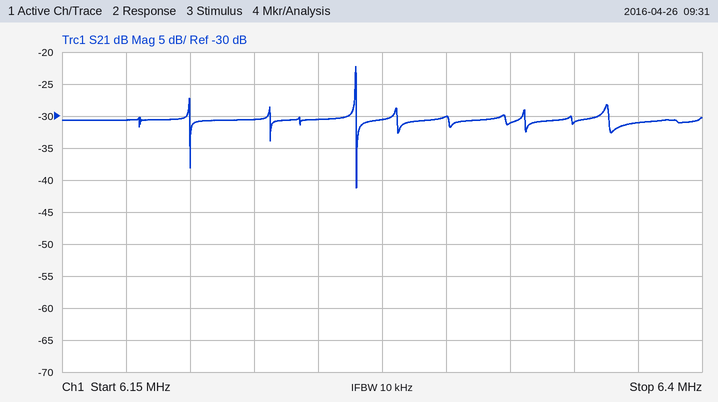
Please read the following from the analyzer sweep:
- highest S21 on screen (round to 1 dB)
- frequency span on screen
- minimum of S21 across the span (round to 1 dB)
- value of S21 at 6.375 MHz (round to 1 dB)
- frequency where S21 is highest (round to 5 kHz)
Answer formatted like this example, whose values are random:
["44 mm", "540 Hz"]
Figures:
["-22 dB", "250 kHz", "-41 dB", "-31 dB", "6.265 MHz"]
